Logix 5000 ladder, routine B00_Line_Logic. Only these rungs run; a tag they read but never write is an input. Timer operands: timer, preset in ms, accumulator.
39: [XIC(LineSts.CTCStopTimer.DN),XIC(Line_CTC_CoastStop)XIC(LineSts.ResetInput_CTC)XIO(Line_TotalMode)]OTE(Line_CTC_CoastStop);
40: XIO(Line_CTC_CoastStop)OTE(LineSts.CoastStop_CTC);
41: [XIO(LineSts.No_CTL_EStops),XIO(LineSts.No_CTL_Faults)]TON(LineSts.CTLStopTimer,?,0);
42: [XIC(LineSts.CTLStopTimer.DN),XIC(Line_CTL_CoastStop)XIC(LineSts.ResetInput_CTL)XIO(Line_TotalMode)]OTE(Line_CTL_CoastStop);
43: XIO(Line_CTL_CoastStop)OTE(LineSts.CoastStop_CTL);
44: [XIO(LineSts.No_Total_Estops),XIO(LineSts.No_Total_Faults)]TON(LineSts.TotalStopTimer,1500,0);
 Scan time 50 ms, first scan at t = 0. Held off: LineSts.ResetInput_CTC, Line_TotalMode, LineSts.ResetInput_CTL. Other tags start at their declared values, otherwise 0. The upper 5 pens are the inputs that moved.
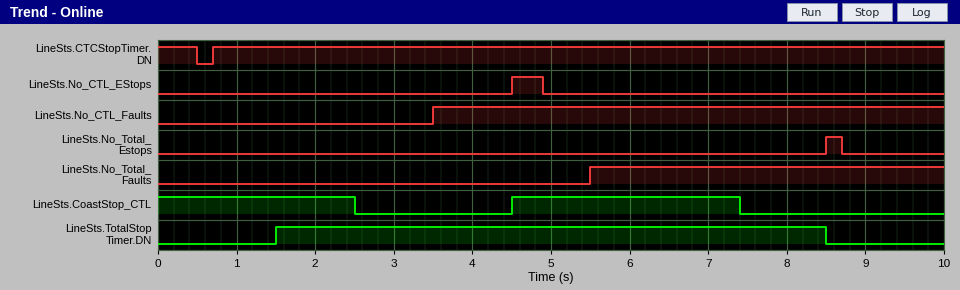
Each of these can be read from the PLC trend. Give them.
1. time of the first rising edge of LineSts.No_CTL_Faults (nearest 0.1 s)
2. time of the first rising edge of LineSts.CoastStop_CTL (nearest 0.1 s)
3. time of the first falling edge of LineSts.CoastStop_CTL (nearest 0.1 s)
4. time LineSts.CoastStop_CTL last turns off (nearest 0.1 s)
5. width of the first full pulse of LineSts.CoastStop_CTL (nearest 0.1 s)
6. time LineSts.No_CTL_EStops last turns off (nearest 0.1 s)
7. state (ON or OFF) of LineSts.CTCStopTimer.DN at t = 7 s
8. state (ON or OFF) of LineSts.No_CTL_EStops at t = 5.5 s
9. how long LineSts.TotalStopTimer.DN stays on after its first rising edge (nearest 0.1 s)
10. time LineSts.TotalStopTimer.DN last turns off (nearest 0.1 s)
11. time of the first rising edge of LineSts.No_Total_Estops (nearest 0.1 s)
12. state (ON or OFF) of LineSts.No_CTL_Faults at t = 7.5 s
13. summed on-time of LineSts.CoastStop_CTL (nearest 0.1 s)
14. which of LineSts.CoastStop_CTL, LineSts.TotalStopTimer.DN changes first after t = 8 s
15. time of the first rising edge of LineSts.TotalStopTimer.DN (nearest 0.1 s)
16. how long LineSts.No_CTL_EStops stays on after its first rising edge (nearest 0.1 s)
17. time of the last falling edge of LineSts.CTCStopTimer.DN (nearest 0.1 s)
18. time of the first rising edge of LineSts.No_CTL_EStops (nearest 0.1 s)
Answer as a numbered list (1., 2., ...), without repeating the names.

1. 3.5 s
2. 4.5 s
3. 2.5 s
4. 7.4 s
5. 2.9 s
6. 4.9 s
7. ON
8. OFF
9. 7.0 s
10. 8.5 s
11. 8.5 s
12. ON
13. 5.4 s
14. LineSts.TotalStopTimer.DN
15. 1.5 s
16. 0.4 s
17. 0.5 s
18. 4.5 s
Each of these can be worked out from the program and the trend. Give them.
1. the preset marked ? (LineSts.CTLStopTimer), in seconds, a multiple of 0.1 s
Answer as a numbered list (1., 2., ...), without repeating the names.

1. 2.5 s
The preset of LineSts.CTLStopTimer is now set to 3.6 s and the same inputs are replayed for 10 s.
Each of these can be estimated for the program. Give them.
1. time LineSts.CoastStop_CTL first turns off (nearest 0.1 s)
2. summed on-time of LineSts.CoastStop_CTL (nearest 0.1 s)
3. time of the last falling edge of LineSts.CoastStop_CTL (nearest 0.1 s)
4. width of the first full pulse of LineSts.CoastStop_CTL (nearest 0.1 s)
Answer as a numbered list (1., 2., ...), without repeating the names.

1. 3.6 s
2. 7.6 s
3. 8.5 s
4. 4.0 s
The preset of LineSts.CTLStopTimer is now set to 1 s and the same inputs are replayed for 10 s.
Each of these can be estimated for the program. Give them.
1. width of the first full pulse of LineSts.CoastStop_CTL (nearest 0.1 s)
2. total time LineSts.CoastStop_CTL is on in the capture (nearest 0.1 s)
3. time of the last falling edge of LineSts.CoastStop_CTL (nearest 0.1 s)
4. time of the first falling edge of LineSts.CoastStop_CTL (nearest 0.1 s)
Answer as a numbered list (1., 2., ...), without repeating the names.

1. 1.4 s
2. 2.4 s
3. 5.9 s
4. 1.0 s
